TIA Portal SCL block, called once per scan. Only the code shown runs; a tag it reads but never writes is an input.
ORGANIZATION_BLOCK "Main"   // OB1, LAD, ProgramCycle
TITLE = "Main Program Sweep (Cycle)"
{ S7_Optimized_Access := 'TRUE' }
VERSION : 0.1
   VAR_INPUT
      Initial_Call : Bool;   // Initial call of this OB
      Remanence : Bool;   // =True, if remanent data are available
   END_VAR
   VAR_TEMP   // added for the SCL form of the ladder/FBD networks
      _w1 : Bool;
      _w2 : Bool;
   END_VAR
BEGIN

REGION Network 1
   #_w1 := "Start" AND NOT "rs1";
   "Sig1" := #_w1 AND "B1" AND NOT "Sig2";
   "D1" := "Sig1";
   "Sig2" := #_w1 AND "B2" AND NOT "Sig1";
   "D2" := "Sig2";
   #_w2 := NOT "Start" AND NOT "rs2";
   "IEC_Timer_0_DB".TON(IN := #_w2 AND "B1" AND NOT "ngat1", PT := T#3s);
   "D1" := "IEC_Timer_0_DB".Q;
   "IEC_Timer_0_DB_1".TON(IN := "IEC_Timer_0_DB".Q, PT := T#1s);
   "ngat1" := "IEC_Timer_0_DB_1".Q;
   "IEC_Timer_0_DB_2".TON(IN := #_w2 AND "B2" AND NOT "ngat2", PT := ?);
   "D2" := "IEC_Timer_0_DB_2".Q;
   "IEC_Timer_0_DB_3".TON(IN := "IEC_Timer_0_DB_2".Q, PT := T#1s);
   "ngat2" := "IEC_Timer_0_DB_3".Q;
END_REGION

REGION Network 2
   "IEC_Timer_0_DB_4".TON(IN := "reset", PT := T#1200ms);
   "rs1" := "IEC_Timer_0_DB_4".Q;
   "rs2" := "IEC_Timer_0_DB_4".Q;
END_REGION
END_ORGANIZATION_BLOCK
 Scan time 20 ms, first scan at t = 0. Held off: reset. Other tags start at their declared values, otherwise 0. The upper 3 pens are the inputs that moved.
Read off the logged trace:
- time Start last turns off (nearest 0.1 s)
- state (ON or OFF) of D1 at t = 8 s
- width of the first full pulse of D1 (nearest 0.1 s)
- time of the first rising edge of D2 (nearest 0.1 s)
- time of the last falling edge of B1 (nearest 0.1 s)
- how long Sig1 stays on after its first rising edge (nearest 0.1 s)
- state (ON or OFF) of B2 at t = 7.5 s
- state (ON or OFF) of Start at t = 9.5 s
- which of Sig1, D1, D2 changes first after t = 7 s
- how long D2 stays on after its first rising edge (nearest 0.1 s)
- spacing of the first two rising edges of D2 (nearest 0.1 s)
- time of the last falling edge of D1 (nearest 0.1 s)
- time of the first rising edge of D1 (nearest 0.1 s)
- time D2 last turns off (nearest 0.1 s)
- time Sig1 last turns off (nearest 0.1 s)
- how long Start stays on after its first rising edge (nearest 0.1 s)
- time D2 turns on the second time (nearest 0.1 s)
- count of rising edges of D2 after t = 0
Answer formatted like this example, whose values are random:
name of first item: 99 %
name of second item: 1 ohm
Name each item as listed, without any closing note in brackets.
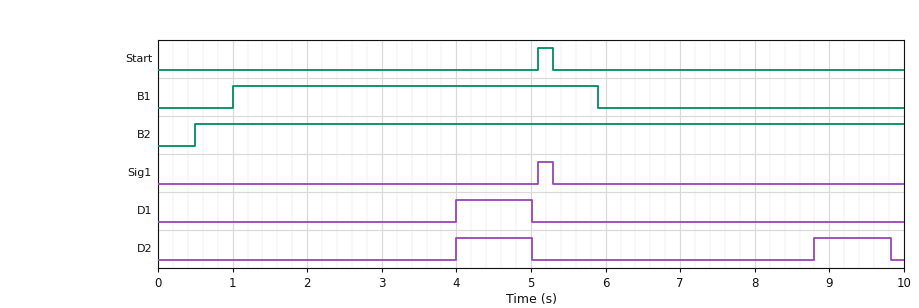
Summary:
time Start last turns off: 5.3 s
state (ON or OFF) of D1 at t = 8 s: OFF
width of the first full pulse of D1: 1.0 s
time of the first rising edge of D2: 4.0 s
time of the last falling edge of B1: 5.9 s
how long Sig1 stays on after its first rising edge: 0.2 s
state (ON or OFF) of B2 at t = 7.5 s: ON
state (ON or OFF) of Start at t = 9.5 s: OFF
which of Sig1, D1, D2 changes first after t = 7 s: D2
how long D2 stays on after its first rising edge: 1.0 s
spacing of the first two rising edges of D2: 4.8 s
time of the last falling edge of D1: 5.0 s
time of the first rising edge of D1: 4.0 s
time D2 last turns off: 9.8 s
time Sig1 last turns off: 5.3 s
how long Start stays on after its first rising edge: 0.2 s
time D2 turns on the second time: 8.8 s
count of rising edges of D2 after t = 0: 2
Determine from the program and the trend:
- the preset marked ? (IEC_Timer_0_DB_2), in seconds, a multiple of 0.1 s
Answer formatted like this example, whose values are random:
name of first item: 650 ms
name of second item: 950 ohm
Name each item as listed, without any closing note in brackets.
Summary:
the preset marked ? (IEC_Timer_0_DB_2), in seconds, a multiple of 0.1 s: 3.5 s
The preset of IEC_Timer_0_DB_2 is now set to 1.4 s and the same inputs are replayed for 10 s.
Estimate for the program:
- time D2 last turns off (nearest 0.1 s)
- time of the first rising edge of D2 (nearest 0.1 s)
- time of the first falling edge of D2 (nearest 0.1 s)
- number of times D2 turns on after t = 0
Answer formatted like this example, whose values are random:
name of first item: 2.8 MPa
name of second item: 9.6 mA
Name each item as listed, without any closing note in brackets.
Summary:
time D2 last turns off: 7.7 s
time of the first rising edge of D2: 1.9 s
time of the first falling edge of D2: 2.9 s
number of times D2 turns on after t = 0: 4
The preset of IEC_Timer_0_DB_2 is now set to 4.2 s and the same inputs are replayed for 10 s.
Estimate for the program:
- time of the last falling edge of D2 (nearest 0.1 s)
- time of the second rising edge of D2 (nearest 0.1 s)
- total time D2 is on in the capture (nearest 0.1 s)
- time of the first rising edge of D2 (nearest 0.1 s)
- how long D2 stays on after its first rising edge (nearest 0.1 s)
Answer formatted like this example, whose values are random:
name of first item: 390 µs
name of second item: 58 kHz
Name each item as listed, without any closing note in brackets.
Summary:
time of the last falling edge of D2: 5.1 s
time of the second rising edge of D2: 9.5 s
total time D2 is on in the capture: 0.9 s
time of the first rising edge of D2: 4.7 s
how long D2 stays on after its first rising edge: 0.4 s
